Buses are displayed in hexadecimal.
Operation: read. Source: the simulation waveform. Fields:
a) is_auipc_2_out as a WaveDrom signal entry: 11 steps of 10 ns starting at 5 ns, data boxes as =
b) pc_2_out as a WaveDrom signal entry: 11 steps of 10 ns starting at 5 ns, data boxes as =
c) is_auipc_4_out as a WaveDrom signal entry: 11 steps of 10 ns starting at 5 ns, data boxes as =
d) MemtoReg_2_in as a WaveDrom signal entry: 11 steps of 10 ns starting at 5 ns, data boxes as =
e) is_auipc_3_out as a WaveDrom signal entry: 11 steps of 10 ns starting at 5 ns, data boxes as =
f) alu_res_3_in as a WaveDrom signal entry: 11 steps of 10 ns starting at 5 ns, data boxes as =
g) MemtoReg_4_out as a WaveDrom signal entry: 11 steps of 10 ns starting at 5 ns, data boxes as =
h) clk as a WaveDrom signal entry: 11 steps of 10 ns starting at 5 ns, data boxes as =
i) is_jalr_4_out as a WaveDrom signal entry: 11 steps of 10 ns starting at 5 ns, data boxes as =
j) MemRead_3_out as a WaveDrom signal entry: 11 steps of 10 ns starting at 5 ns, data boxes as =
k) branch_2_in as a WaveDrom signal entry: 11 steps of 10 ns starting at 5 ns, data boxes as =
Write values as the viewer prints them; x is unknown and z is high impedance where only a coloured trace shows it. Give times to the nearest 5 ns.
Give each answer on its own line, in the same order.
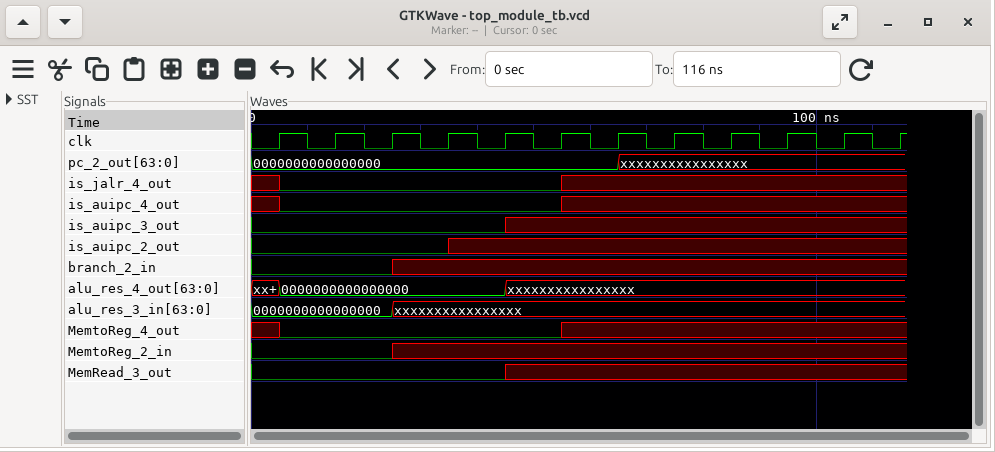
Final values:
{name: 'is_auipc_2_out', wave: '0..x.......'}
{name: 'pc_2_out', wave: '=.....x....', data: '0000000000000000'}
{name: 'is_auipc_4_out', wave: '0....x.....'}
{name: 'MemtoReg_2_in', wave: '0.x........'}
{name: 'is_auipc_3_out', wave: '0...x......'}
{name: 'alu_res_3_in', wave: '=.x........', data: '0000000000000000'}
{name: 'MemtoReg_4_out', wave: '0....x.....'}
{name: 'clk', wave: 'p..........'}
{name: 'is_jalr_4_out', wave: '0....x.....'}
{name: 'MemRead_3_out', wave: '0...x......'}
{name: 'branch_2_in', wave: '0.x........'}
